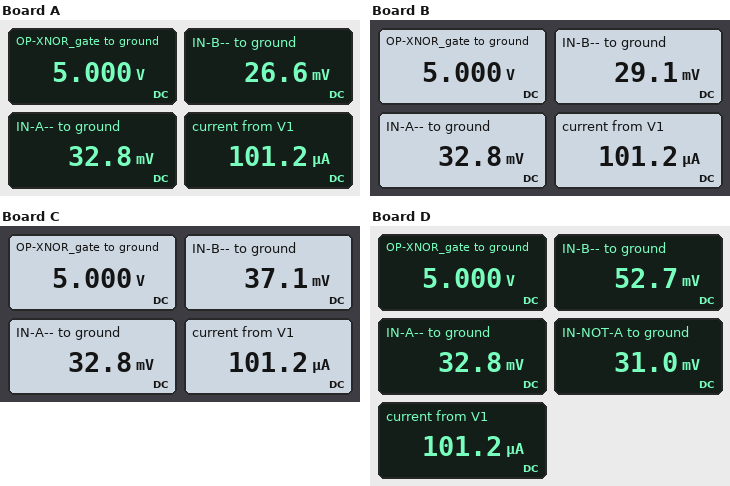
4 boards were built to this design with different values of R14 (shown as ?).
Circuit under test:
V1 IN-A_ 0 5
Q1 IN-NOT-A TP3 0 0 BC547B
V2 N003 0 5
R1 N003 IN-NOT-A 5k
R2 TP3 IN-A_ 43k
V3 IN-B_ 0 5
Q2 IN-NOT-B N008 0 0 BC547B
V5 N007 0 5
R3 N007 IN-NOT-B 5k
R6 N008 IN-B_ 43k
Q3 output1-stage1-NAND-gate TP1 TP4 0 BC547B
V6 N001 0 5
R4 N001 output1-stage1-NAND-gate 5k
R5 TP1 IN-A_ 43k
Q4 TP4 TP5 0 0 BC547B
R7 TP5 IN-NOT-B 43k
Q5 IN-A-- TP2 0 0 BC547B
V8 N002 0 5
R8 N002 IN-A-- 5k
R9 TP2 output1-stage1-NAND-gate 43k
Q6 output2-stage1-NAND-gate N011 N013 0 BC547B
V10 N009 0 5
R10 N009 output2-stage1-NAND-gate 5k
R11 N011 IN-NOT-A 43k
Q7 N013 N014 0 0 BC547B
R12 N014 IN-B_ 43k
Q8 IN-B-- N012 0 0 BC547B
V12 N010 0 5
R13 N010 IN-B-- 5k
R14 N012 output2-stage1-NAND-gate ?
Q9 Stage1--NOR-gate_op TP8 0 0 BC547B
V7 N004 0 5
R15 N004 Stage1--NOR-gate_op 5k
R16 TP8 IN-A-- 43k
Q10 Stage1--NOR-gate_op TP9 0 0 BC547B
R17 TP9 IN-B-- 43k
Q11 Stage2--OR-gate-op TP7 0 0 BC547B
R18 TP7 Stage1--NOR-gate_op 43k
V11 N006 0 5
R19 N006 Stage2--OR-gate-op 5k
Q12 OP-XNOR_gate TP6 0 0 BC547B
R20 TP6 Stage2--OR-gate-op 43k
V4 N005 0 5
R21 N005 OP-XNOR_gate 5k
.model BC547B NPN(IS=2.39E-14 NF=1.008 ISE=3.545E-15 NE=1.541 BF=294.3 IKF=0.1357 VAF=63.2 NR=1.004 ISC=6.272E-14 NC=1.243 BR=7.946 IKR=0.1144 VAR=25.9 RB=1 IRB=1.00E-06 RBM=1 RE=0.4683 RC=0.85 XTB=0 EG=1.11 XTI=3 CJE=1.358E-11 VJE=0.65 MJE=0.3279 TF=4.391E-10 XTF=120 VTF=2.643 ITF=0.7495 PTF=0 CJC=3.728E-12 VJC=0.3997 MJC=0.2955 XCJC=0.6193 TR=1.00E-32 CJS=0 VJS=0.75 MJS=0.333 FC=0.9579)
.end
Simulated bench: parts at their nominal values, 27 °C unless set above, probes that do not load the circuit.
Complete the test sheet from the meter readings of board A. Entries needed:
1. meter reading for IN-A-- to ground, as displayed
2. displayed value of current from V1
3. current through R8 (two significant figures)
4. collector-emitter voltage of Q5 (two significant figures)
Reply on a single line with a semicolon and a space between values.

32.8 mV; 101.2 µA; 990 µA; 33 mV
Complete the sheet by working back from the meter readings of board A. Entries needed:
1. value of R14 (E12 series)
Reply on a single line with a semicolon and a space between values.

27 kΩ
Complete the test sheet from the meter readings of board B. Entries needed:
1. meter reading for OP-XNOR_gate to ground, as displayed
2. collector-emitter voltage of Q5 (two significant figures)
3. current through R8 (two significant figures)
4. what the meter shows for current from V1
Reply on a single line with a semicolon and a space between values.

5.000 V; 33 mV; 990 µA; 101.2 µA
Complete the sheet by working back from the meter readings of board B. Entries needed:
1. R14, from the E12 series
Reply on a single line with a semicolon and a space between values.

33 kΩ
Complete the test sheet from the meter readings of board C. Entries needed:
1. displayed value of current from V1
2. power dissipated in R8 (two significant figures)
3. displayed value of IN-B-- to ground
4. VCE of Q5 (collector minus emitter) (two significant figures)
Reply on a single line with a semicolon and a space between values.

101.2 µA; 4.9 mW; 37.1 mV; 33 mV
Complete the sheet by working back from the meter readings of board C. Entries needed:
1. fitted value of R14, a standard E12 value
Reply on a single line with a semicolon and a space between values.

56 kΩ
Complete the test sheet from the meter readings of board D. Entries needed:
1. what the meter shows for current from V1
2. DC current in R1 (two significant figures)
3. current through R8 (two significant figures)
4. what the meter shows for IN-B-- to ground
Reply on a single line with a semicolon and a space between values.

101.2 µA; 990 µA; 990 µA; 52.7 mV
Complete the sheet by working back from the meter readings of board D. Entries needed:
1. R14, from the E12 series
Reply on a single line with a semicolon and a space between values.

120 kΩ
